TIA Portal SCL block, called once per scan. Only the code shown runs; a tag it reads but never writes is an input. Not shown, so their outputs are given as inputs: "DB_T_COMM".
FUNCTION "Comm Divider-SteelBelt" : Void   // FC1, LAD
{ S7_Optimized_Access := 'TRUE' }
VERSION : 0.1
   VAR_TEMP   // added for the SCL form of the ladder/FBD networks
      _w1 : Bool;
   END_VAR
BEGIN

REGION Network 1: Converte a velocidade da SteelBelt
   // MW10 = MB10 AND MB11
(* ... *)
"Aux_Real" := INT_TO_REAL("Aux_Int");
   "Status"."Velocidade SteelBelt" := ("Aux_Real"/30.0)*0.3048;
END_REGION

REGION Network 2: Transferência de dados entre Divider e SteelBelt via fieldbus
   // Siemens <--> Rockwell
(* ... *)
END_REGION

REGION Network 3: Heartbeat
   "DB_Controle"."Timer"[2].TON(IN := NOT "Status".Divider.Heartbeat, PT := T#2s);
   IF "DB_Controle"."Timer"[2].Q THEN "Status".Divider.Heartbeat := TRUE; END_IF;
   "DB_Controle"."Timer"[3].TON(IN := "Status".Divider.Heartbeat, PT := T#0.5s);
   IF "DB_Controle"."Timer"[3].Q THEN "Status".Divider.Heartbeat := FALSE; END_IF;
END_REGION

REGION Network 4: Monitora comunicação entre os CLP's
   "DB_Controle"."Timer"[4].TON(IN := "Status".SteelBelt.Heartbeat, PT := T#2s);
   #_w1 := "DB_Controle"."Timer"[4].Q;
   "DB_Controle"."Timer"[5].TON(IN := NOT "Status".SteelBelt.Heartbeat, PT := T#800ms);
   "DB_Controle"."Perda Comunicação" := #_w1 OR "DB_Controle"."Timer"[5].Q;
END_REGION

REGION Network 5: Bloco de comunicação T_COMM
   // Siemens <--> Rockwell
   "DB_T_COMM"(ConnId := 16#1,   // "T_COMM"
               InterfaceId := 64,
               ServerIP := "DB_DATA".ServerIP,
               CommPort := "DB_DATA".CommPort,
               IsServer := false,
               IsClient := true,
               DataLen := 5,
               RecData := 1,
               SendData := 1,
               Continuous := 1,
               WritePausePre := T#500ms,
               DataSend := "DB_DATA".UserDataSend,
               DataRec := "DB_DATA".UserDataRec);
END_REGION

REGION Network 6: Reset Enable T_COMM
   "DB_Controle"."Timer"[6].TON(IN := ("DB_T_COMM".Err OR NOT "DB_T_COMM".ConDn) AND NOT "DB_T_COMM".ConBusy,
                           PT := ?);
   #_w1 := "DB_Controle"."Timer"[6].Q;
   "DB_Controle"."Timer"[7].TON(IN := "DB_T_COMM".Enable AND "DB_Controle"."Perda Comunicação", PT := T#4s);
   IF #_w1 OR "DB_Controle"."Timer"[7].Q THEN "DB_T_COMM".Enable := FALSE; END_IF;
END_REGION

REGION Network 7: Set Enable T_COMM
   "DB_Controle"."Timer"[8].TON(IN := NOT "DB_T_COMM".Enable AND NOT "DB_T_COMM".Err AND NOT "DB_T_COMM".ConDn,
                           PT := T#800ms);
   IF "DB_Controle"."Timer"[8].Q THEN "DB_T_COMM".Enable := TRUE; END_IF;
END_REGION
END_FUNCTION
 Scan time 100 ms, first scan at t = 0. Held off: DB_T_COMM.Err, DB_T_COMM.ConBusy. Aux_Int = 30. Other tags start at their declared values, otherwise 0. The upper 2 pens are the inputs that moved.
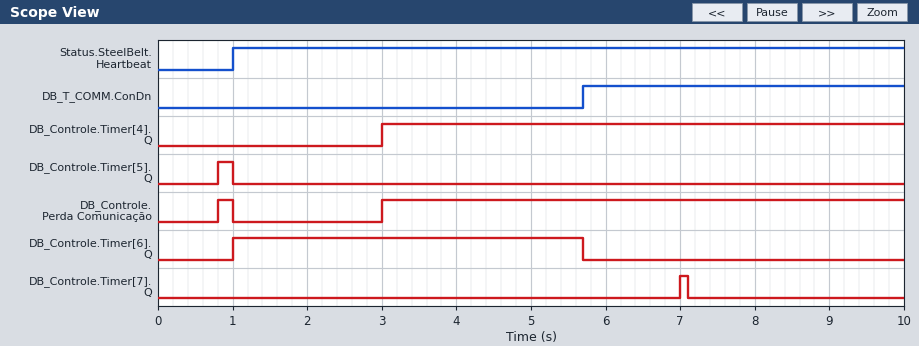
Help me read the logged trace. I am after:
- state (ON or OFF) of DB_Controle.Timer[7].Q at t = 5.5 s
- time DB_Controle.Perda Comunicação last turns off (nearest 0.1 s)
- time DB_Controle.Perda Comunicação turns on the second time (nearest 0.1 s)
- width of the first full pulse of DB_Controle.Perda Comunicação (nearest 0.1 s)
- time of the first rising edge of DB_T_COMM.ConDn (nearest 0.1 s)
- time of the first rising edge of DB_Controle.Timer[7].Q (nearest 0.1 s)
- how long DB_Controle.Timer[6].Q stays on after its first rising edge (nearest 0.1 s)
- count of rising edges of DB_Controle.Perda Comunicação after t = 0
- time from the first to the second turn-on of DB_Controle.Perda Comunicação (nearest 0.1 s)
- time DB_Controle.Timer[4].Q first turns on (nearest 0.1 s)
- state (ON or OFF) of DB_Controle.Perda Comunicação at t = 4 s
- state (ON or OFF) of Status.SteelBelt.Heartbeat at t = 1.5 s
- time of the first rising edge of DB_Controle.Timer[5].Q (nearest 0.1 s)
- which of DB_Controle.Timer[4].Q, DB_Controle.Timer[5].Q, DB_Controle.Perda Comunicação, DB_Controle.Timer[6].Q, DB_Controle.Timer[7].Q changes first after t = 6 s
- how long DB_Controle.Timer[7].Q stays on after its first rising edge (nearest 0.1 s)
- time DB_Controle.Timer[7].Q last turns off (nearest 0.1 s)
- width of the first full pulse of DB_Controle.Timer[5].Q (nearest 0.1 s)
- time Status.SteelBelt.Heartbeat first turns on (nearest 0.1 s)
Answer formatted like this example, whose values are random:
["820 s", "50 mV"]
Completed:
["OFF", "1.0 s", "3.0 s", "0.2 s", "5.7 s", "7.0 s", "4.7 s", "2", "2.2 s", "3.0 s", "ON", "ON", "0.8 s", "DB_Controle.Timer[7].Q", "0.1 s", "7.1 s", "0.2 s", "1.0 s"]
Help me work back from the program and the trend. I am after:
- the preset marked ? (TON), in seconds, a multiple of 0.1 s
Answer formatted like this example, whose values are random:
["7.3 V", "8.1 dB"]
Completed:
["1.0 s"]
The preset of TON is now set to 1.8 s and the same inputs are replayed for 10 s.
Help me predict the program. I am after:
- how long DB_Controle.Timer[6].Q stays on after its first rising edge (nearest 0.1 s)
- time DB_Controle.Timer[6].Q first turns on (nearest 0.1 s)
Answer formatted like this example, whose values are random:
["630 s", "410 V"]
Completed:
["3.9 s", "1.8 s"]
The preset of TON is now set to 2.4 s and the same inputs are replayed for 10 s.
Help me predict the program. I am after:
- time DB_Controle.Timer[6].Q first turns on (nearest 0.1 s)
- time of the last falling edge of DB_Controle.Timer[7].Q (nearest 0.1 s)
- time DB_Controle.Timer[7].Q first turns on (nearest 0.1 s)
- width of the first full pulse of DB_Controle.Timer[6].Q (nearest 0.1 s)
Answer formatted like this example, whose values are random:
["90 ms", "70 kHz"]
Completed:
["2.4 s", "7.4 s", "7.3 s", "3.3 s"]
